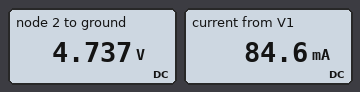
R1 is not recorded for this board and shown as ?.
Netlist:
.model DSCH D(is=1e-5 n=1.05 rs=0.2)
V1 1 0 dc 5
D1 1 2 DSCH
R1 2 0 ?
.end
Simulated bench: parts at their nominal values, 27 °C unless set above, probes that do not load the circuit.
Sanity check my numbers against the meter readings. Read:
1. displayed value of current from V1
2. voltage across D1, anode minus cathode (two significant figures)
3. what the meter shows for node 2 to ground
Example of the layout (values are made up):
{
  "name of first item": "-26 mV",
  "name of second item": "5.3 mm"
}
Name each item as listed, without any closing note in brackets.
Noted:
{
  "displayed value of current from V1": "84.6 mA",
  "voltage across D1, anode minus cathode": "260 mV",
  "what the meter shows for node 2 to ground": "4.737 V"
}
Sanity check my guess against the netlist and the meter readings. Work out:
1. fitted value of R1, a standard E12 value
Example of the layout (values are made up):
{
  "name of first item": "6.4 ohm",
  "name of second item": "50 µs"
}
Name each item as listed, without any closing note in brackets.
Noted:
{
  "fitted value of R1, a standard E12 value": "56 Ω"
}
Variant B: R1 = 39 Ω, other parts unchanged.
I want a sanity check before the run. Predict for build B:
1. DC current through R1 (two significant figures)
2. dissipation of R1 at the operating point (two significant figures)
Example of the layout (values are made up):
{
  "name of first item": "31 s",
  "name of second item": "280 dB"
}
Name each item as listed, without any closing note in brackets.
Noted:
{
  "DC current through R1": "120 mA",
  "dissipation of R1 at the operating point": "570 mW"
}
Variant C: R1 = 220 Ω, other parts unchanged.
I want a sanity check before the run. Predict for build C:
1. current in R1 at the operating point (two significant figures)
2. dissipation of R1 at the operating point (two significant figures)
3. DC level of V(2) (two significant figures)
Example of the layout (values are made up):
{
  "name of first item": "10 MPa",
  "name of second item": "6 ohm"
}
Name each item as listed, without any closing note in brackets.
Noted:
{
  "current in R1 at the operating point": "22 mA",
  "dissipation of R1 at the operating point": "100 mW",
  "DC level of V(2)": "4.8 V"
}
